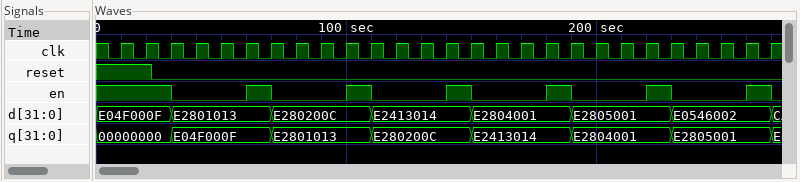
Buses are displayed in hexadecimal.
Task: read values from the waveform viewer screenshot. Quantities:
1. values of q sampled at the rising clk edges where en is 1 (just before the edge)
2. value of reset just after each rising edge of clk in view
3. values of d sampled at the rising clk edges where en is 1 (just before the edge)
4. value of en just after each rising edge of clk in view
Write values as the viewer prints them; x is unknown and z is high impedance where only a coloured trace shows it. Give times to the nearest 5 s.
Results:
00000000, 00000000, 00000000, E04F000F, E2801013, E280200C, E2413014, E2804001, E2805001
1 1 0 0 0 0 0 0 0 0 0 0 0 0 0 0 0 0 0 0 0 0 0 0 0 0 0
E04F000F, E04F000F, E04F000F, E2801013, E280200C, E2413014, E2804001, E2805001, E0546002
1 1 0 0 0 1 0 0 0 1 0 0 0 1 0 0 0 1 0 0 0 1 0 0 0 1 0
